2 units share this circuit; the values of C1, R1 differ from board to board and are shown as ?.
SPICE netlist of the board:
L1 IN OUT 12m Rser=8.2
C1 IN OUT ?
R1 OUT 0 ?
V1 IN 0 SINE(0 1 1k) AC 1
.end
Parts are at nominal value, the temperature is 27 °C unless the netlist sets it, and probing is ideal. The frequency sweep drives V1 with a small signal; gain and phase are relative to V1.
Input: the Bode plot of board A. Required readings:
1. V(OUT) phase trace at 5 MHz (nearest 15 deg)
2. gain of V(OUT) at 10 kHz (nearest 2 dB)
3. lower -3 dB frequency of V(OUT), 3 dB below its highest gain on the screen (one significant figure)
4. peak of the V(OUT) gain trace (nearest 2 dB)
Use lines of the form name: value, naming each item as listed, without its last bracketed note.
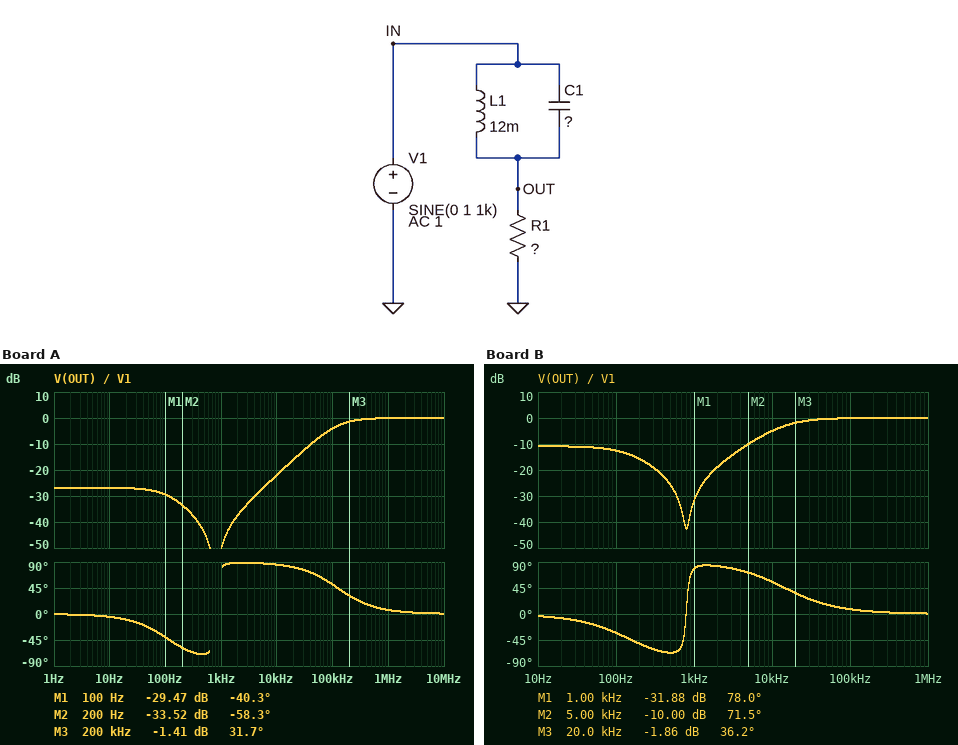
V(OUT) phase trace at 5 MHz: 0 deg
gain of V(OUT) at 10 kHz: -22 dB
lower -3 dB frequency of V(OUT), 3 dB below its highest gain on the screen: 100 kHz
peak of the V(OUT) gain trace: 0 dB
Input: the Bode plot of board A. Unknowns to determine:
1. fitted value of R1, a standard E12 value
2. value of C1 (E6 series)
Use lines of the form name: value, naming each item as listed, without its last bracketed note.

fitted value of R1, a standard E12 value: 0.39 Ω
value of C1: 3.3 µF
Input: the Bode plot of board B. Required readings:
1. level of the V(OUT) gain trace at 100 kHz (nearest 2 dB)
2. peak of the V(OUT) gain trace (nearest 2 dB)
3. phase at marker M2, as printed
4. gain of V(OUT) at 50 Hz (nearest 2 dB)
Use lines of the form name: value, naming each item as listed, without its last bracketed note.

level of the V(OUT) gain trace at 100 kHz: 0 dB
peak of the V(OUT) gain trace: 0 dB
phase at marker M2, as printed: 71.5 deg
gain of V(OUT) at 50 Hz: -12 dB
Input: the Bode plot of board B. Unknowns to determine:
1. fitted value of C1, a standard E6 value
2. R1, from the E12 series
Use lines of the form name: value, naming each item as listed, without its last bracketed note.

fitted value of C1, a standard E6 value: 3.3 µF
R1, from the E12 series: 3.3 Ω
